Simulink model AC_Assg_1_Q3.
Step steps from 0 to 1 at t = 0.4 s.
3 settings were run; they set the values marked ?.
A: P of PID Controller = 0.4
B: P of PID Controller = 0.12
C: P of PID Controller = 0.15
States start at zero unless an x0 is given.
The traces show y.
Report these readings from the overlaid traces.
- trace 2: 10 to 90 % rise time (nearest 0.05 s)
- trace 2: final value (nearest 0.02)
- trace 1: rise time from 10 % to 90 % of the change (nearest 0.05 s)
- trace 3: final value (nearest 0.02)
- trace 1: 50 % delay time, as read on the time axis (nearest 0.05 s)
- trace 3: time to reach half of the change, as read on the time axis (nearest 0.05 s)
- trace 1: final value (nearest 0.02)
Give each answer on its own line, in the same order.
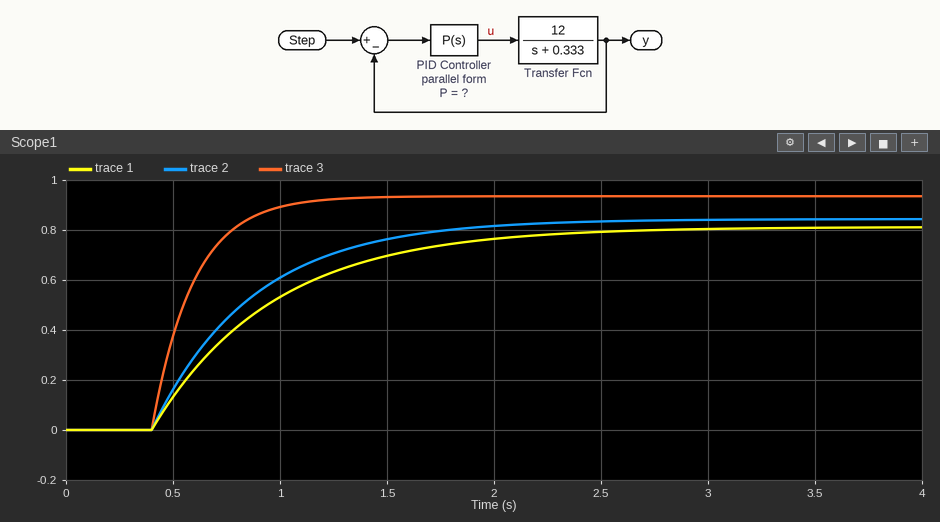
1.05 s
0.84
1.25 s
0.94
0.80 s
0.55 s
0.82
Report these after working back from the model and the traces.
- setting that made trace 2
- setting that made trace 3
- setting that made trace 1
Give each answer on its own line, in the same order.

C
A
B
